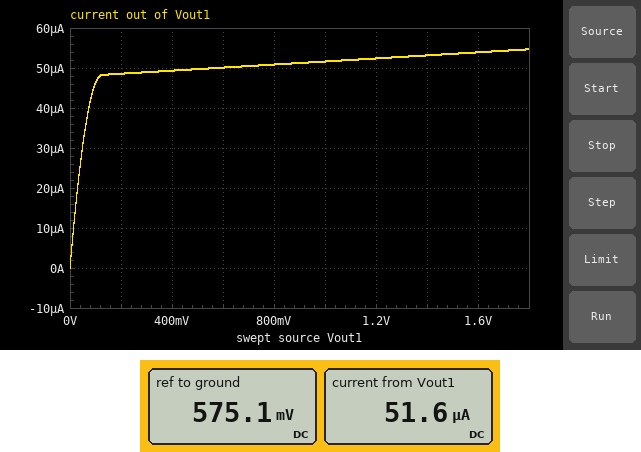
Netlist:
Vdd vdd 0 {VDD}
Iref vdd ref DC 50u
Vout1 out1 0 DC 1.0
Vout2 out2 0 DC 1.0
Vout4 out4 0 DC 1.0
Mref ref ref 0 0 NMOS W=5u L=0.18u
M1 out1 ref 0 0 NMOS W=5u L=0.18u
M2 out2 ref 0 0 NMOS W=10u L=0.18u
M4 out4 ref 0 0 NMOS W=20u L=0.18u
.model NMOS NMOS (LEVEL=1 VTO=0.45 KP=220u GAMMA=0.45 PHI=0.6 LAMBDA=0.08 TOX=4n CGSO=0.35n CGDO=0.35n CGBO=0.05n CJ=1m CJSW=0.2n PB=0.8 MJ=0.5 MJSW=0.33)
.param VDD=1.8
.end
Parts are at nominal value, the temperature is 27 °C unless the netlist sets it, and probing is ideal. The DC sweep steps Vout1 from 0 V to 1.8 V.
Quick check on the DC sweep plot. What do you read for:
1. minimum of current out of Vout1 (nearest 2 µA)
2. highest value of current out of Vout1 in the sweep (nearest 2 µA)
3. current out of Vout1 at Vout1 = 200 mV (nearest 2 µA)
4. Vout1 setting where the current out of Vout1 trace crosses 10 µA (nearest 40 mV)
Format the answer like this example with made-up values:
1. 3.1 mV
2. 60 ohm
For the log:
1. 0 A
2. 54 µA
3. 48 µA
4. 0 V
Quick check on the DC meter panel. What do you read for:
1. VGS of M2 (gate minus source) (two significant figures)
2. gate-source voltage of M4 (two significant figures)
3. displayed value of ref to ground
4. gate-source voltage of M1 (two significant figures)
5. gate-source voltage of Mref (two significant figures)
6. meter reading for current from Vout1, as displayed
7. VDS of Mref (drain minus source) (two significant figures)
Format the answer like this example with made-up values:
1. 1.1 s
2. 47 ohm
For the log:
1. 580 mV
2. 580 mV
3. 575.1 mV
4. 580 mV
5. 580 mV
6. 51.6 µA
7. 580 mV
